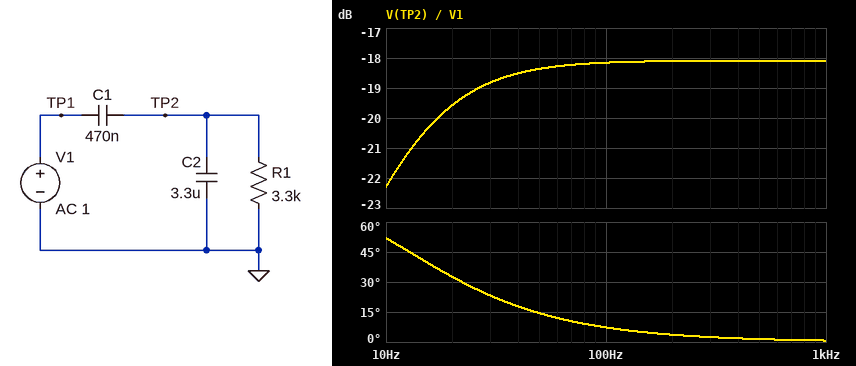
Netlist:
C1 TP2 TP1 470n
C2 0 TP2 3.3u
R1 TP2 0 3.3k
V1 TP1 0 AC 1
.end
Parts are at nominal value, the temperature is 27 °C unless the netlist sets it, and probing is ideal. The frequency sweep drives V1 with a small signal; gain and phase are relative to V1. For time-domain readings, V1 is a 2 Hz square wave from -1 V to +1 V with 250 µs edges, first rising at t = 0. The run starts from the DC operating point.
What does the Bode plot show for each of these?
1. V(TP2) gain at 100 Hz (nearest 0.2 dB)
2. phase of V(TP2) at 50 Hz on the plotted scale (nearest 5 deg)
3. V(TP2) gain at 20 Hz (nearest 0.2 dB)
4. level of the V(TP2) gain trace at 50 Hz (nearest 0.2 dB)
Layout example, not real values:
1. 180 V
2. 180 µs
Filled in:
1. -18.2 dB
2. 15 deg
3. -19.6 dB
4. -18.4 dB
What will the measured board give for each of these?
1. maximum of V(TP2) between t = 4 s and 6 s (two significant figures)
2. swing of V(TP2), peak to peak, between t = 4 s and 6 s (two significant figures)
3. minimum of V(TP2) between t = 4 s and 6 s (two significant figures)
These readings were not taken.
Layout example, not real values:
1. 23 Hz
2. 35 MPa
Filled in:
1. 250 mV
2. 490 mV
3. -250 mV
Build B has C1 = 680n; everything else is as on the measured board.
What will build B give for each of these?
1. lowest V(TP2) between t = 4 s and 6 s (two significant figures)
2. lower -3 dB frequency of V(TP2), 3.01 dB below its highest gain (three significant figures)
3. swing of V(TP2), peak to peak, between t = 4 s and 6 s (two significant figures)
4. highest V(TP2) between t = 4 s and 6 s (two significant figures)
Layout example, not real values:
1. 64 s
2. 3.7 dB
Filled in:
1. -340 mV
2. 12.1 Hz
3. 680 mV
4. 340 mV
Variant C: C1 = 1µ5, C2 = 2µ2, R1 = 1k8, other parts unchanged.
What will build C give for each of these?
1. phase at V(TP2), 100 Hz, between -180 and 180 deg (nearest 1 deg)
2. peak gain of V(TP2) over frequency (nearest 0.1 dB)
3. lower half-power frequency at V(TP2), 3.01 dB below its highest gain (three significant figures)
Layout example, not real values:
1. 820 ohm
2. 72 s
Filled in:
1. 13 deg
2. -7.8 dB
3. 23.9 Hz
